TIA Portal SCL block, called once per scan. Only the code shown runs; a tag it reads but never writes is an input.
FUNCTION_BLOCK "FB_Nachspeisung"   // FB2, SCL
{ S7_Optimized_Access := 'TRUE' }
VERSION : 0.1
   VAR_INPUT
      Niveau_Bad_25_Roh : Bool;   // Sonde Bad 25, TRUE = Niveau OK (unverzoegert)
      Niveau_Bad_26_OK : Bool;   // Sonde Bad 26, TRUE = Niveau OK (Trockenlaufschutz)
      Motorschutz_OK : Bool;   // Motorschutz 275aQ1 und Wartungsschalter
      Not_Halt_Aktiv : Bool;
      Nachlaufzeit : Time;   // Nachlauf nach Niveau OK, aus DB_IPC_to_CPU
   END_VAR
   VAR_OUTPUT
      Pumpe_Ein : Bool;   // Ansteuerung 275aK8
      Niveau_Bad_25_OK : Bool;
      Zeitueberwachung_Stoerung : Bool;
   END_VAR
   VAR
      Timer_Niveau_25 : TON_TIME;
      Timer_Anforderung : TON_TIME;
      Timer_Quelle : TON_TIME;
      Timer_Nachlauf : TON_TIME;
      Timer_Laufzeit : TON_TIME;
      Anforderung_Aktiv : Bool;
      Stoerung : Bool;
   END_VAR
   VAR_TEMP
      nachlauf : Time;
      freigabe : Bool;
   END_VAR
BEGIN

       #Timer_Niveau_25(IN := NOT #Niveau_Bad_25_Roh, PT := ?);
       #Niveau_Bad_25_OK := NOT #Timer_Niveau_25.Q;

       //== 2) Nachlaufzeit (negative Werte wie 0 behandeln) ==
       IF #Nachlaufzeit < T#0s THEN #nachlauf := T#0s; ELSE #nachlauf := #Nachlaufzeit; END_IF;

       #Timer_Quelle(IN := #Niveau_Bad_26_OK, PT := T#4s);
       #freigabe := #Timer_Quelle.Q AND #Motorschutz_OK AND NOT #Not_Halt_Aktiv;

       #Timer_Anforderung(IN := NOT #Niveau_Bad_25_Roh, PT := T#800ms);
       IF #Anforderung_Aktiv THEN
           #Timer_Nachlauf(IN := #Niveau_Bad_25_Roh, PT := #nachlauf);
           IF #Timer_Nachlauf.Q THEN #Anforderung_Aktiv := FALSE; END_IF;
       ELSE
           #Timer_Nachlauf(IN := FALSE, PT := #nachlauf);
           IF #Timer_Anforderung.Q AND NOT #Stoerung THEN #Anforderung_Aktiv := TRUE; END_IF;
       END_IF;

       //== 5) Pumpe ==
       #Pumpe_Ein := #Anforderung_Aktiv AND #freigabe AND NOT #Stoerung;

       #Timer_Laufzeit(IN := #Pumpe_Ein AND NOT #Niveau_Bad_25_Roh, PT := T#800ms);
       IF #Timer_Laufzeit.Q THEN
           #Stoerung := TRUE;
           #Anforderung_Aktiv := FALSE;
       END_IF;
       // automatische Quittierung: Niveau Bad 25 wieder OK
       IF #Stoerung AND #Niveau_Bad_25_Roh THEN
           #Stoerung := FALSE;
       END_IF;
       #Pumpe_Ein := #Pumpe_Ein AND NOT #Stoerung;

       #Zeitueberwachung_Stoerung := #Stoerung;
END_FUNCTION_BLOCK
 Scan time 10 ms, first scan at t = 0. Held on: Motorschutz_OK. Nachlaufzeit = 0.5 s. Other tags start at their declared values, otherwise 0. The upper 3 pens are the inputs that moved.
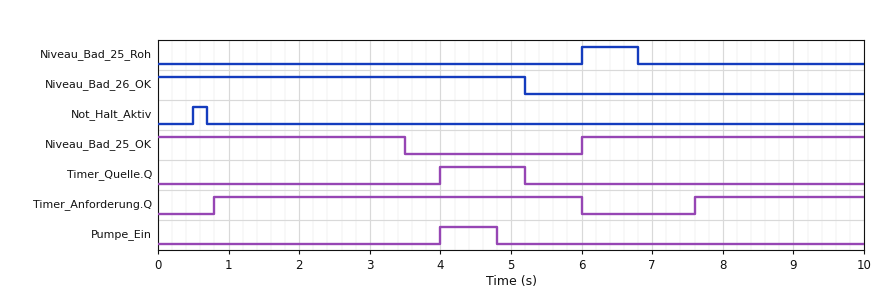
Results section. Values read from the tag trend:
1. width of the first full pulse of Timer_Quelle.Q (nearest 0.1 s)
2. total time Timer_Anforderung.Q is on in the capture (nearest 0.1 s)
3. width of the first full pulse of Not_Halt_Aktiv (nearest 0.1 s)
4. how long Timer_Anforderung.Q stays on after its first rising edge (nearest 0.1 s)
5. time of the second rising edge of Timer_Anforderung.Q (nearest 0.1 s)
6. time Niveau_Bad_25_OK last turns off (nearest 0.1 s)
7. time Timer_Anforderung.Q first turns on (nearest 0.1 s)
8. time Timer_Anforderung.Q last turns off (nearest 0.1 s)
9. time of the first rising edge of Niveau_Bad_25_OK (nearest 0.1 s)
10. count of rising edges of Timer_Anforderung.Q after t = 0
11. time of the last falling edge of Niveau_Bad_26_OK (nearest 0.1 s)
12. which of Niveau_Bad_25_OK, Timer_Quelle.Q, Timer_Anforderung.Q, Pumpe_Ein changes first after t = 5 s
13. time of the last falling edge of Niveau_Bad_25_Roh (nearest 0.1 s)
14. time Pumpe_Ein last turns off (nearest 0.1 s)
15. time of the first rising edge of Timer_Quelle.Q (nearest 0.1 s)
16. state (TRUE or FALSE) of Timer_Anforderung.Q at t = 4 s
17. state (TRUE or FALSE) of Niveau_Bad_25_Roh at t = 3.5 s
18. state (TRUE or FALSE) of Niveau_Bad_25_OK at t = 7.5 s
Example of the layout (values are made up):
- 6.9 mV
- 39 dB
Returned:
- 1.2 s
- 7.6 s
- 0.2 s
- 5.2 s
- 7.6 s
- 3.5 s
- 0.8 s
- 6.0 s
- 6.0 s
- 2
- 5.2 s
- Timer_Quelle.Q
- 6.8 s
- 4.8 s
- 4.0 s
- TRUE
- FALSE
- TRUE
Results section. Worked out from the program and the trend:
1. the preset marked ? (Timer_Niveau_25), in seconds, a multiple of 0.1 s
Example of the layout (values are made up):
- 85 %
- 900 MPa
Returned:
- 3.5 s
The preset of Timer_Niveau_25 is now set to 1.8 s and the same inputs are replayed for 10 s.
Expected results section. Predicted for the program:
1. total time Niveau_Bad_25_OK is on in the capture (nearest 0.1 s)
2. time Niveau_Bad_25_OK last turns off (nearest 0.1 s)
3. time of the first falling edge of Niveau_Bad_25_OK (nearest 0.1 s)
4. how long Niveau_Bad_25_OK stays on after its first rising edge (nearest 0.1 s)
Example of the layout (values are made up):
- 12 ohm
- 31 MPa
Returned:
- 4.4 s
- 8.6 s
- 1.8 s
- 2.6 s
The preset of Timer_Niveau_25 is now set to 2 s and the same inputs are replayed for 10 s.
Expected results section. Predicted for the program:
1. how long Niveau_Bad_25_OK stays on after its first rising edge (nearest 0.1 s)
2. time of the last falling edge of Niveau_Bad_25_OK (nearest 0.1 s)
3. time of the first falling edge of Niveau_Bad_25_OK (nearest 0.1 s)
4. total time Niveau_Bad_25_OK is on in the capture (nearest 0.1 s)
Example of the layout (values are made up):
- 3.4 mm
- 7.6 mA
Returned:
- 2.8 s
- 8.8 s
- 2.0 s
- 4.8 s
